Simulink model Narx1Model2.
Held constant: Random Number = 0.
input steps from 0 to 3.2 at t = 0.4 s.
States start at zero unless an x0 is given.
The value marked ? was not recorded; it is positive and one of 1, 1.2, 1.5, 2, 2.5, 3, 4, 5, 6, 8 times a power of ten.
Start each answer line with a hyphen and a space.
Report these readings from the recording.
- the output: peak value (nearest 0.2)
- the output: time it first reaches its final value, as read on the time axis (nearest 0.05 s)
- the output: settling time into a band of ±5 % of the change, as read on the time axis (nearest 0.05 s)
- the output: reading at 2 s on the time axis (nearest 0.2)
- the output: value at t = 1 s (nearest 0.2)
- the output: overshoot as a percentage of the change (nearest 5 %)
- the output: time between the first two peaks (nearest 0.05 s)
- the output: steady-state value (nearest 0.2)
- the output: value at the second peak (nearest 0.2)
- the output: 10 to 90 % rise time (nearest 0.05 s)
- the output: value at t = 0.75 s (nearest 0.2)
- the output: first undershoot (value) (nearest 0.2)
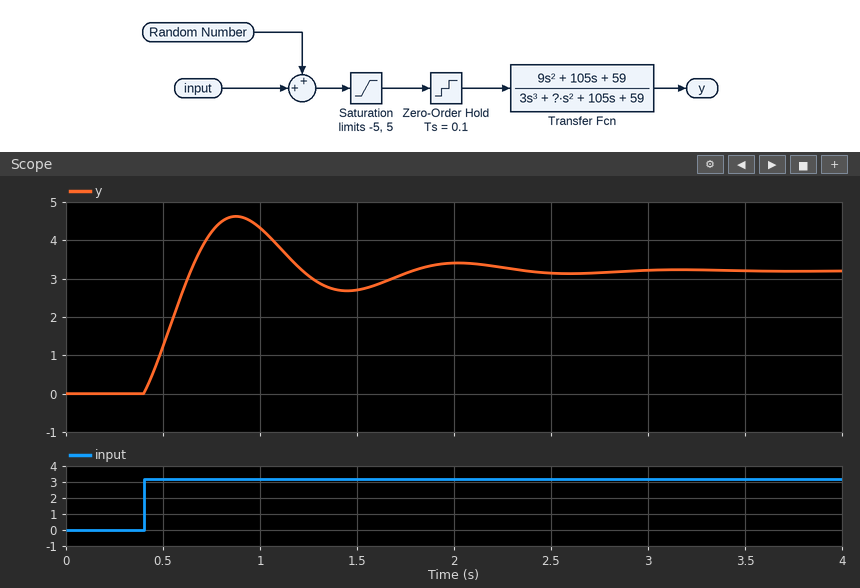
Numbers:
- 4.6
- 0.65 s
- 2.15 s
- 3.4
- 4.4
- 45 %
- 1.15 s
- 3.2
- 3.4
- 0.20 s
- 4.2
- 2.6
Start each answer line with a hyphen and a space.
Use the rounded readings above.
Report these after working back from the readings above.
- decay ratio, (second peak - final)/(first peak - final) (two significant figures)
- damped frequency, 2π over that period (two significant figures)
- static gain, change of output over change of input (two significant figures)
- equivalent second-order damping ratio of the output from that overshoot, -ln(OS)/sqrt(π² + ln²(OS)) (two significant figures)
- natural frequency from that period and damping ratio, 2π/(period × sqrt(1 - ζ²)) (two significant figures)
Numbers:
- 0.14
- 5.5 rad/s
- 1.0
- 0.25
- 5.6 rad/s
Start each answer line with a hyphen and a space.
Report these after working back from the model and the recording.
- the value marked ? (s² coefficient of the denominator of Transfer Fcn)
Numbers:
- 12
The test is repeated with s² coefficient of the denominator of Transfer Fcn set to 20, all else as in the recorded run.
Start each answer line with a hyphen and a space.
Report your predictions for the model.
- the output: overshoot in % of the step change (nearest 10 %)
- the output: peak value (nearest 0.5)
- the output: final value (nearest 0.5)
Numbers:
- 20 %
- 4.0
- 3.0
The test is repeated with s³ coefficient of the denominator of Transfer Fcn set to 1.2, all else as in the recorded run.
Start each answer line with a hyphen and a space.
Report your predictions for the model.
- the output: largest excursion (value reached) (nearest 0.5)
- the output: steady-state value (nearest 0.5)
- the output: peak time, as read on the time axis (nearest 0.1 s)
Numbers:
- 4.0
- 3.0
- 0.7 s
